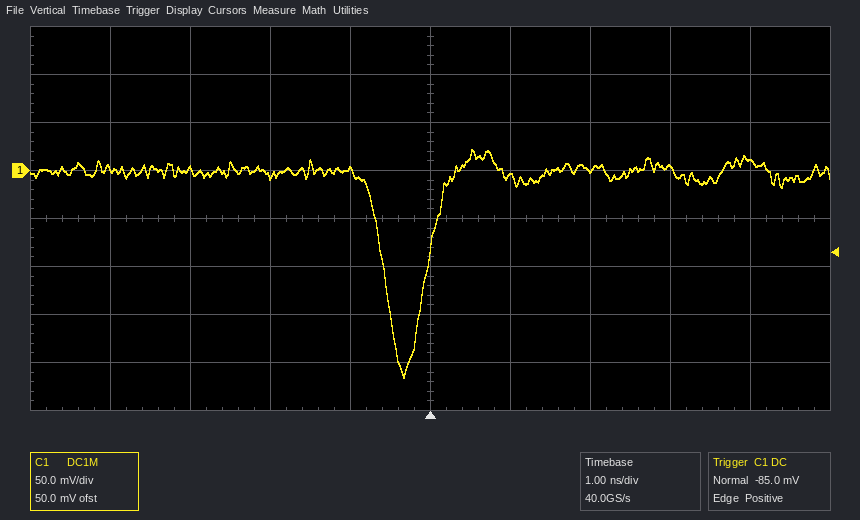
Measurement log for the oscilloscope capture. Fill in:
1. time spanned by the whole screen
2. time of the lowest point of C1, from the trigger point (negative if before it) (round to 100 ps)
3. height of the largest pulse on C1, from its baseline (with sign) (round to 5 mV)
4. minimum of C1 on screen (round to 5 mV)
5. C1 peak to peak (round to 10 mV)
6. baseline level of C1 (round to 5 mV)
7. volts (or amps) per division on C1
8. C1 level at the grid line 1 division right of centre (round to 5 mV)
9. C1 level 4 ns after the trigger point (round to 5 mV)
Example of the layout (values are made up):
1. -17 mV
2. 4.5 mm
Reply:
1. 10 ns
2. -300 ps
3. -215 mV
4. -215 mV
5. 240 mV
6. 0 mV
7. 50 mV
8. -5 mV
9. 10 mV
